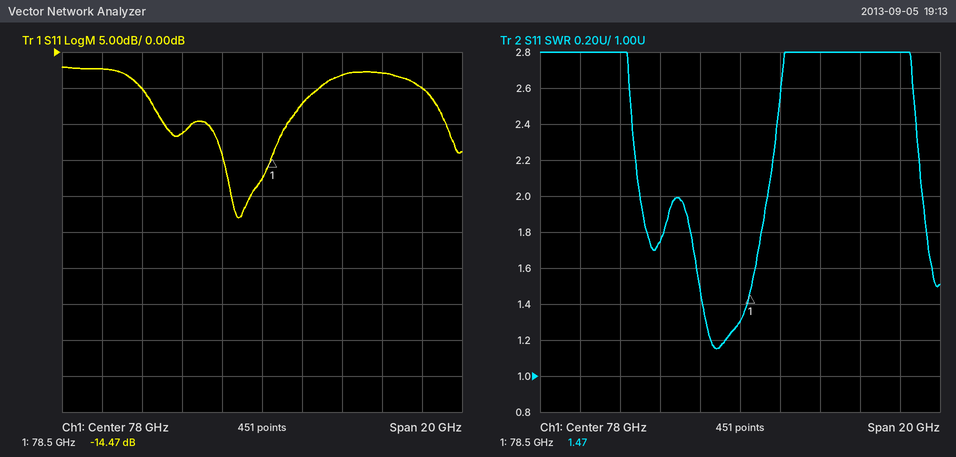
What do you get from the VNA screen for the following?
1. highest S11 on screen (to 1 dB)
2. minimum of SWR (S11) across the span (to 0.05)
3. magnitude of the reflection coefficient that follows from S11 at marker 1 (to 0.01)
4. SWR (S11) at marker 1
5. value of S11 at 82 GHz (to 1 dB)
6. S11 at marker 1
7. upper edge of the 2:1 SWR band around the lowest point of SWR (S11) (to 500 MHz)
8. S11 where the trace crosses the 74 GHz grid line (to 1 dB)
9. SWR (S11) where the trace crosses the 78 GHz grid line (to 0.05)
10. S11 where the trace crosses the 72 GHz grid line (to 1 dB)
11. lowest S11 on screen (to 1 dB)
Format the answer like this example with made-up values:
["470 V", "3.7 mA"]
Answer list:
["-2 dB", "1.15", "0.19", "1.47", "-3 dB", "-14.47 dB", "79.5 GHz", "-11 dB", "1.30", "-5 dB", "-23 dB"]
